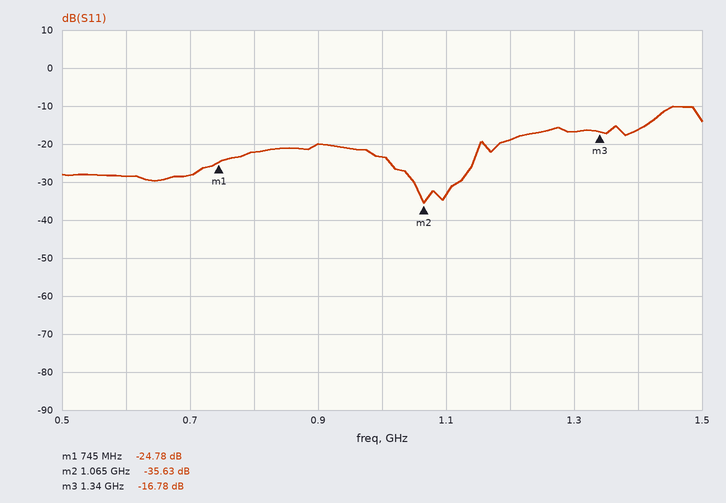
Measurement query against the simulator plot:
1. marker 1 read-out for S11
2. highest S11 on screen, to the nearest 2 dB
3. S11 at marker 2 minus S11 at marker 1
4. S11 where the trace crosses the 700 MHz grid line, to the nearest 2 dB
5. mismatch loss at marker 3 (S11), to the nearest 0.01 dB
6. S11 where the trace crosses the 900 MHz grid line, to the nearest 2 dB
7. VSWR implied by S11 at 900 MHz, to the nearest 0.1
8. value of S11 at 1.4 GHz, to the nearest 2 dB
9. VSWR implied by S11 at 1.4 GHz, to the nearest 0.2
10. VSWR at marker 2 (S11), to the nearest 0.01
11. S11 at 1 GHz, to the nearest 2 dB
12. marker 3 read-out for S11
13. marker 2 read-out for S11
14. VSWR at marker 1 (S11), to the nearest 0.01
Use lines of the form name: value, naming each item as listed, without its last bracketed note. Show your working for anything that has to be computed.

marker 1 read-out for S11: -24.78 dB
highest S11 on screen, to the nearest 2 dB: -10 dB
S11 at marker 2 minus S11 at marker 1: -35.63 − (-24.78) = -10.85 dB
S11 where the trace crosses the 700 MHz grid line, to the nearest 2 dB: -28 dB
mismatch loss at marker 3 (S11), to the nearest 0.01 dB: −10 log10(1 − 10^(-16.78/10)) ≈ 0.09 dB
S11 where the trace crosses the 900 MHz grid line, to the nearest 2 dB: -20 dB
VSWR implied by S11 at 900 MHz, to the nearest 0.1: |Γ| = 10^(-20/20) = 0.1000; VSWR = (1 + 0.1000)/(1 − 0.1000) ≈ 1.2
value of S11 at 1.4 GHz, to the nearest 2 dB: -16 dB
VSWR implied by S11 at 1.4 GHz, to the nearest 0.2: |Γ| = 10^(-16/20) = 0.1585; VSWR = (1 + 0.1585)/(1 − 0.1585) ≈ 1.4
VSWR at marker 2 (S11), to the nearest 0.01: (1 + 0.0165)/(1 − 0.0165) ≈ 1.03
S11 at 1 GHz, to the nearest 2 dB: -24 dB
marker 3 read-out for S11: -16.78 dB
marker 2 read-out for S11: -35.63 dB
VSWR at marker 1 (S11), to the nearest 0.01: (1 + 0.0577)/(1 − 0.0577) ≈ 1.12
